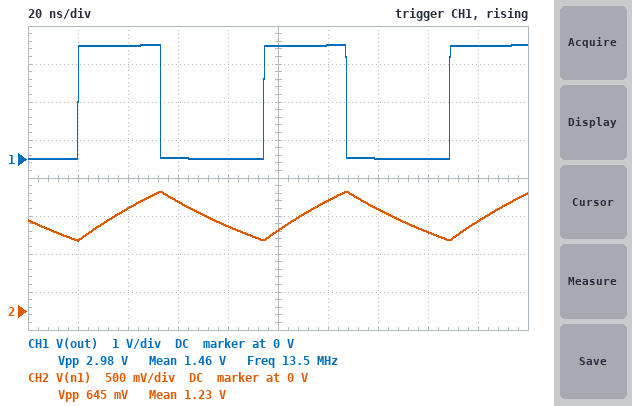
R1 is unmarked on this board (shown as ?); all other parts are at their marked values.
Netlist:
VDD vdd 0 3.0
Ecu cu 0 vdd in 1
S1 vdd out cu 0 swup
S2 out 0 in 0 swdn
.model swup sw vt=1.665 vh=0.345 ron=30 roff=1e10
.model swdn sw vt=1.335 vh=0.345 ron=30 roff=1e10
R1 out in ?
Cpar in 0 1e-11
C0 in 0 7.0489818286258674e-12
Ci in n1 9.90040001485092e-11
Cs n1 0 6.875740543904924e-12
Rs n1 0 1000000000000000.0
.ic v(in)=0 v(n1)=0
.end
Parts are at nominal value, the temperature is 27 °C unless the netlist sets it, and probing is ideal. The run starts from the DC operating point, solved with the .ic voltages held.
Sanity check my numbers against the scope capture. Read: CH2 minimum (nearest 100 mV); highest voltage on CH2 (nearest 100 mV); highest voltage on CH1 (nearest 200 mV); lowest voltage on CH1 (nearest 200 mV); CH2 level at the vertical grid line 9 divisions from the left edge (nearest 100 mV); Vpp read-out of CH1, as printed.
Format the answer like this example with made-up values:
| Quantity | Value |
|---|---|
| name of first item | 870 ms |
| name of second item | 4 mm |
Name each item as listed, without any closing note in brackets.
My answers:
| Quantity | Value |
|---|---|
| CH2 minimum | 900 mV |
| highest voltage on CH2 | 1.6 V |
| highest voltage on CH1 | 3.0 V |
| lowest voltage on CH1 | 0 V |
| CH2 level at the vertical grid line 9 divisions from the left edge | 1.2 V |
| Vpp read-out of CH1, as printed | 2.98 V |
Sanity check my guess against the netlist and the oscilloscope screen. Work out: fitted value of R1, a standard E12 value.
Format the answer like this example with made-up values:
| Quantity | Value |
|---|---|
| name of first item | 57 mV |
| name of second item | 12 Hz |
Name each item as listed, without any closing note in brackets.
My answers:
| Quantity | Value |
|---|---|
| fitted value of R1, a standard E12 value | 3.3 kΩ |
